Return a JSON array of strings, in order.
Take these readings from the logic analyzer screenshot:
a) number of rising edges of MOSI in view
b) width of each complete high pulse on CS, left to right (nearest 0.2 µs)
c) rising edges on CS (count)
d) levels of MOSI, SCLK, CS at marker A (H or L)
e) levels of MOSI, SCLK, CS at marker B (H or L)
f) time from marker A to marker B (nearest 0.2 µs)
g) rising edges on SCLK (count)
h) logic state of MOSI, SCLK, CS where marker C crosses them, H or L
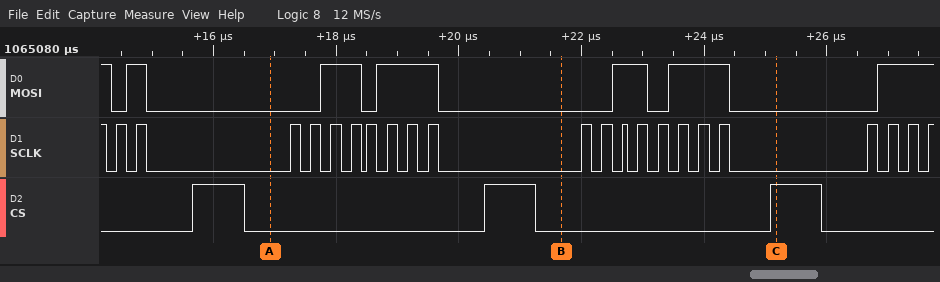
["6", "0.8 µs, 0.8 µs, 0.8 µs", "3", "MOSI=L, SCLK=L, CS=L", "MOSI=L, SCLK=L, CS=L", "4.8 µs", "22", "MOSI=L, SCLK=L, CS=H"]
